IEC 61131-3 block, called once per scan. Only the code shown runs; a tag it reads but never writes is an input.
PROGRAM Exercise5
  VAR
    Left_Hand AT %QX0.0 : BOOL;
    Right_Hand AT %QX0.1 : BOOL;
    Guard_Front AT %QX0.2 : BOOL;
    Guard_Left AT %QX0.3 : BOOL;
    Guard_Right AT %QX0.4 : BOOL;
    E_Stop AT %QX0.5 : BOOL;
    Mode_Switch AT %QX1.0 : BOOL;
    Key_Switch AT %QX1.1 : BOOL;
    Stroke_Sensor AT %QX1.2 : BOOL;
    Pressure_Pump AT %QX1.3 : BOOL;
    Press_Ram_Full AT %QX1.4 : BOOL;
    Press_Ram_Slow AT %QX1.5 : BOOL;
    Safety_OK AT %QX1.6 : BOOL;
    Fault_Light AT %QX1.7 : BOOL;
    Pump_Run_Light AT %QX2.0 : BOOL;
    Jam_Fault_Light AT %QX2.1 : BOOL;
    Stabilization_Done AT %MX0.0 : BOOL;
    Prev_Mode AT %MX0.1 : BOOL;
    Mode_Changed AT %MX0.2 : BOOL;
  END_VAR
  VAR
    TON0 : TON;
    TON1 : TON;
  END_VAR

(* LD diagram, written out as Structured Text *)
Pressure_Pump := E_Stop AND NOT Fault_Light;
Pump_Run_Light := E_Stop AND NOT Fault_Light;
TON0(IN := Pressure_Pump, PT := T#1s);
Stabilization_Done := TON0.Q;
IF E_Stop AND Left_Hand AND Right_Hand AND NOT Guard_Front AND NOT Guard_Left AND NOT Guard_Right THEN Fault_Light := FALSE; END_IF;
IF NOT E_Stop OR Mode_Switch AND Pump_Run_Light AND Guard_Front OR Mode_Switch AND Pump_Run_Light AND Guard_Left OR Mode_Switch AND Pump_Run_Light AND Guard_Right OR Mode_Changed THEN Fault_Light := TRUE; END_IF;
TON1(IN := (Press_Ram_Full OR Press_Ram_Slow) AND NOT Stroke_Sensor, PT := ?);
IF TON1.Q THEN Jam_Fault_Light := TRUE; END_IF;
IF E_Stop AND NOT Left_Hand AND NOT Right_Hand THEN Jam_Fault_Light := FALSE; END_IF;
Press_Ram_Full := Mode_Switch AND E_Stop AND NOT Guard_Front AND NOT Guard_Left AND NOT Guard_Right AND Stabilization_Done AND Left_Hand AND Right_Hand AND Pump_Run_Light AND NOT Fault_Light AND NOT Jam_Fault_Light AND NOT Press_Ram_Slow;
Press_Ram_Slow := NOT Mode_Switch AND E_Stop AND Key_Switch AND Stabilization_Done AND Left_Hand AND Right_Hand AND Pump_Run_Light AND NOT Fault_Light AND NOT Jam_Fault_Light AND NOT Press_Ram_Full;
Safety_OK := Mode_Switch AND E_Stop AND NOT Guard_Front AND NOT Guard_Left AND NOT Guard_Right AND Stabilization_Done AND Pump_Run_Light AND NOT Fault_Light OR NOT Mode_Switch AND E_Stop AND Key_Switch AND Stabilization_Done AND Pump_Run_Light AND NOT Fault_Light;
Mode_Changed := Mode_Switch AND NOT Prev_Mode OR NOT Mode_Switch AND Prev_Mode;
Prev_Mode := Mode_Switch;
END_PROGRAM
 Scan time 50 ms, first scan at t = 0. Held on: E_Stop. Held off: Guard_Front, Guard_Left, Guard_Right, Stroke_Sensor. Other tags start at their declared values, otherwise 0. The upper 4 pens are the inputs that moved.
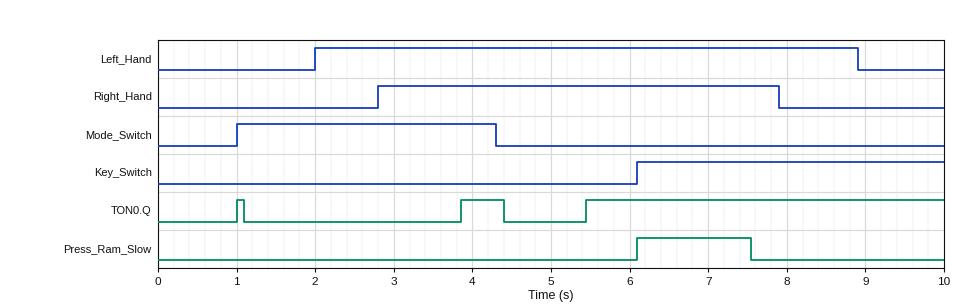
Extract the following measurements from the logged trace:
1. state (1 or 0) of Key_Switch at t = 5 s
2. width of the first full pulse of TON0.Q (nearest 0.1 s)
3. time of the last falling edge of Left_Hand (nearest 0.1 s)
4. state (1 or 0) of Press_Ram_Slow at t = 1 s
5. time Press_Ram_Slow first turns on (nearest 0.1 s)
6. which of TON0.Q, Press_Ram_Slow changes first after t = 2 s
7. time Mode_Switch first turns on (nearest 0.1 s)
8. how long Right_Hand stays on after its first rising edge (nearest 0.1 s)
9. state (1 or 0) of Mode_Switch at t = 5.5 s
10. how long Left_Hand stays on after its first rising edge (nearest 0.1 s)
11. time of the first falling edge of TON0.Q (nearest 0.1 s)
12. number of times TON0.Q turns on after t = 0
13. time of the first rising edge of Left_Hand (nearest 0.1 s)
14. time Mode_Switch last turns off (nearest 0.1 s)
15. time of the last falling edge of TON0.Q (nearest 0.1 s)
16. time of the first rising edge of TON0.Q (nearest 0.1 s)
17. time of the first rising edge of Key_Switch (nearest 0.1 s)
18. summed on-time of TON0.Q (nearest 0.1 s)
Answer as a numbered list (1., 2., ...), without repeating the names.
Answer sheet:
1. 0
2. 0.1 s
3. 8.9 s
4. 0
5. 6.1 s
6. TON0.Q
7. 1.0 s
8. 5.1 s
9. 0
10. 6.9 s
11. 1.1 s
12. 3
13. 2.0 s
14. 4.3 s
15. 4.4 s
16. 1.0 s
17. 6.1 s
18. 5.2 s
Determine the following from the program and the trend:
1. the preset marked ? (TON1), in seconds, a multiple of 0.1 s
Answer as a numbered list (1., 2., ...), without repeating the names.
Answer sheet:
1. 1.4 s
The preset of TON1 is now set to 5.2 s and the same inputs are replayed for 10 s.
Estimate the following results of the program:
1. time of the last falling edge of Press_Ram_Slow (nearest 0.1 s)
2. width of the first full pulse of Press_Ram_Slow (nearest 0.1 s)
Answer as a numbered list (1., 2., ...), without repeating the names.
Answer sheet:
1. 7.9 s
2. 1.8 s
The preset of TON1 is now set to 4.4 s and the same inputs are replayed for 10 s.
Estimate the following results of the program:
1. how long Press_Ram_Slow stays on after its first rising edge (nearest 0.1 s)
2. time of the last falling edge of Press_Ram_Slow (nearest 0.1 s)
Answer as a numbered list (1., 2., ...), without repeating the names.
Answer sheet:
1. 1.8 s
2. 7.9 s
